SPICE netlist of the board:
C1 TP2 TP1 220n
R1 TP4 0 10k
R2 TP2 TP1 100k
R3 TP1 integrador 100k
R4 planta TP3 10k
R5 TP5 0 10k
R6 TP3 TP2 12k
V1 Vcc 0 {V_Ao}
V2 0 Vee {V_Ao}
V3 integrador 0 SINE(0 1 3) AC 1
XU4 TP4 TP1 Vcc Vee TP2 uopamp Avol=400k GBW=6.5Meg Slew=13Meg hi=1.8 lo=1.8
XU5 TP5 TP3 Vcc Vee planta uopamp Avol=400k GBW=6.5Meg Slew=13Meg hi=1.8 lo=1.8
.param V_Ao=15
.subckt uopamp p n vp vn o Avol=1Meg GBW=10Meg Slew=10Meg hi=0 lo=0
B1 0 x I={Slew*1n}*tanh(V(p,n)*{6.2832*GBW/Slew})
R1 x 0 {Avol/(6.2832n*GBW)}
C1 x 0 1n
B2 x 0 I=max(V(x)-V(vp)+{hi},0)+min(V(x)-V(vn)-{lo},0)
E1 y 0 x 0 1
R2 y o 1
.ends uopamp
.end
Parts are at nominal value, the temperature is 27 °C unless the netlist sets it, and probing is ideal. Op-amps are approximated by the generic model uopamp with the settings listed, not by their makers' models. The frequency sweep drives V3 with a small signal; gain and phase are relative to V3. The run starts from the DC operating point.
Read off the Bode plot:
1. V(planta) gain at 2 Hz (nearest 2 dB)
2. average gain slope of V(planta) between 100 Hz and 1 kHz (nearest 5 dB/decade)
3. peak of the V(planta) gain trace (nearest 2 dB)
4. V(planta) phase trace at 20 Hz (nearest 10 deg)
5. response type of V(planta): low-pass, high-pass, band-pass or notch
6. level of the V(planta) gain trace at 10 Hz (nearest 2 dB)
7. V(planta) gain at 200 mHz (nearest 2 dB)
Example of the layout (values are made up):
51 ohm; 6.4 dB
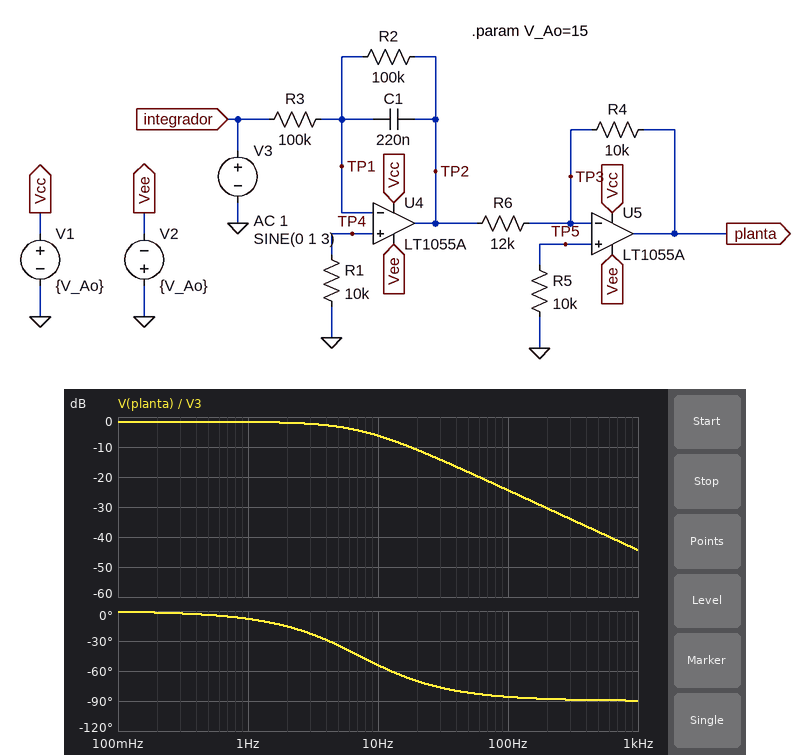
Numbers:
-2 dB; -20 dB/decade; -2 dB; -70 deg; low-pass; -6 dB; -2 dB
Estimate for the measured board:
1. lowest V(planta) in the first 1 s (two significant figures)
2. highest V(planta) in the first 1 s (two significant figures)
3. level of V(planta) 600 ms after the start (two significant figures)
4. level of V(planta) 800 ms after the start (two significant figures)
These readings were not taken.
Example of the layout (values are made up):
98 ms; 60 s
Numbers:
-770 mV; 770 mV; -770 mV; 660 mV
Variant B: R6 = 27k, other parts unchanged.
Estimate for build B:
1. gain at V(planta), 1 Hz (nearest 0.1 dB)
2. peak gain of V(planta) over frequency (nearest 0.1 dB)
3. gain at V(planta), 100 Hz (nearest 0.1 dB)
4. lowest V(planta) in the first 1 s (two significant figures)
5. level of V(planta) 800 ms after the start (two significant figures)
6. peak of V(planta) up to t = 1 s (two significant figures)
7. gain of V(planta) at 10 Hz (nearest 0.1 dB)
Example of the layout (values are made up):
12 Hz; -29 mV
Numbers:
-8.7 dB; -8.6 dB; -31.5 dB; -340 mV; 290 mV; 340 mV; -13.3 dB
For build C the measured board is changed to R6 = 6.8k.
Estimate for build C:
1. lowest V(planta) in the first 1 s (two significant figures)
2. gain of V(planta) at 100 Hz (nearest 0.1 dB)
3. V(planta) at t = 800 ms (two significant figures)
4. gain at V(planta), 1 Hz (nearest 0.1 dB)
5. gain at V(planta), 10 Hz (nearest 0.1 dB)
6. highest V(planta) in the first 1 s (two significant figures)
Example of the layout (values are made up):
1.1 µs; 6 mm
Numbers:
-1.4 V; -19.5 dB; 1.2 V; 3.3 dB; -1.3 dB; 1.4 V
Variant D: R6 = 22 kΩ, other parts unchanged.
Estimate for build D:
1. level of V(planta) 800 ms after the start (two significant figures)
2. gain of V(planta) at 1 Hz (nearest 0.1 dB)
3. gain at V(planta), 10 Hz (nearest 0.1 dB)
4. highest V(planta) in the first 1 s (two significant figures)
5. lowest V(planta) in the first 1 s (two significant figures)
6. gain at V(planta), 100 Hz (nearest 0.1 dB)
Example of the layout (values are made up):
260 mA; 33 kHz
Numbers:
360 mV; -6.9 dB; -11.5 dB; 420 mV; -420 mV; -29.7 dB
